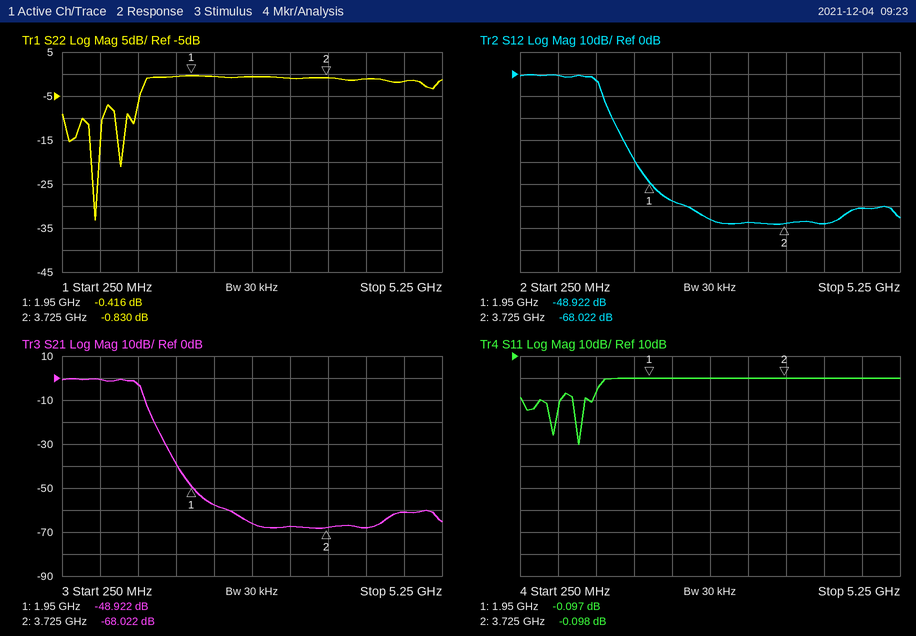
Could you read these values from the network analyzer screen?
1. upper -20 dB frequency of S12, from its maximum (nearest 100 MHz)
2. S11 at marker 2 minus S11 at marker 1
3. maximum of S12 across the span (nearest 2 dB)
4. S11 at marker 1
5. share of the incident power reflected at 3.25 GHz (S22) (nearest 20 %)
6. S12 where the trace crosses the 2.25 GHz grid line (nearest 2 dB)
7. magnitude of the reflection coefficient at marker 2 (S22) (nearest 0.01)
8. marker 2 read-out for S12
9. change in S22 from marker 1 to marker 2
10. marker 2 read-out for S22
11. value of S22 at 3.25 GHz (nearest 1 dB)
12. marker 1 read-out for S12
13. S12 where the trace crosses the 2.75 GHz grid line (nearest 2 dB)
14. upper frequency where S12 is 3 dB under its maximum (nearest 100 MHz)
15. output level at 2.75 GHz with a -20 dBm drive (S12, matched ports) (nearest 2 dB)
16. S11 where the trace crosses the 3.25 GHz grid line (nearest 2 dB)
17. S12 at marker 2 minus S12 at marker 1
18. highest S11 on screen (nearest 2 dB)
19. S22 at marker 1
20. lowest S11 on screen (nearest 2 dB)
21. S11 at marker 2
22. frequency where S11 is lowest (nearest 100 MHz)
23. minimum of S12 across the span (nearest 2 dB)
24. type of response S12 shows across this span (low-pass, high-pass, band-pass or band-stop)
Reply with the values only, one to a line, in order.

1.5 GHz
-0.001 dB
0 dB
-0.097 dB
80 %
-58 dB
0.91
-68.022 dB
-0.414 dB
-0.830 dB
-1 dB
-48.922 dB
-66 dB
1.3 GHz
-86 dBm
0 dB
-19.100 dB
0 dB
-0.416 dB
-30 dB
-0.098 dB
1.0 GHz
-68 dB
low-pass
